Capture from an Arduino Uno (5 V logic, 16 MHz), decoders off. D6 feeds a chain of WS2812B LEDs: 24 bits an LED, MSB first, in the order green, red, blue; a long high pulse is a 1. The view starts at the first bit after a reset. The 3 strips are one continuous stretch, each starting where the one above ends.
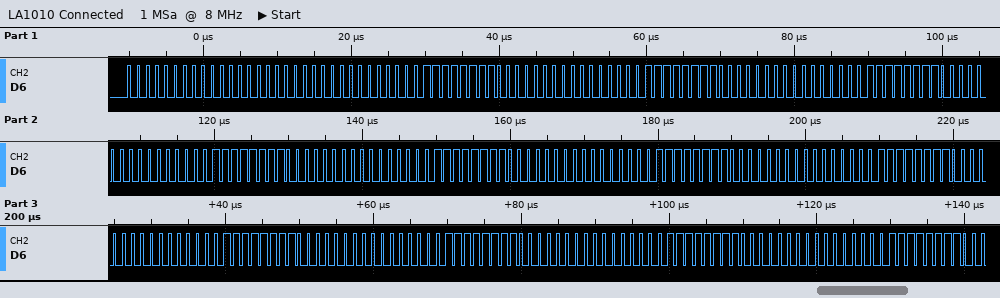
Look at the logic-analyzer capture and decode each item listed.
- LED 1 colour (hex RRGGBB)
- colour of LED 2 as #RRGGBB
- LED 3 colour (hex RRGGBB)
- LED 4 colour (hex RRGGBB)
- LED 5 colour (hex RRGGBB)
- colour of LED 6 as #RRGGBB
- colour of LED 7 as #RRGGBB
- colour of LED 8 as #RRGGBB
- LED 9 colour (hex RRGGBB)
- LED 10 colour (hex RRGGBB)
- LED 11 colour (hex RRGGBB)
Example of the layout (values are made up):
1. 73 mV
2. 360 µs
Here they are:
1. #000000
2. #FF0000
3. #FF0000
4. #FF0000
5. #FF0000
6. #FF0000
7. #FF0000
8. #FF0000
9. #FF0000
10. #FF0000
11. #FF0000
